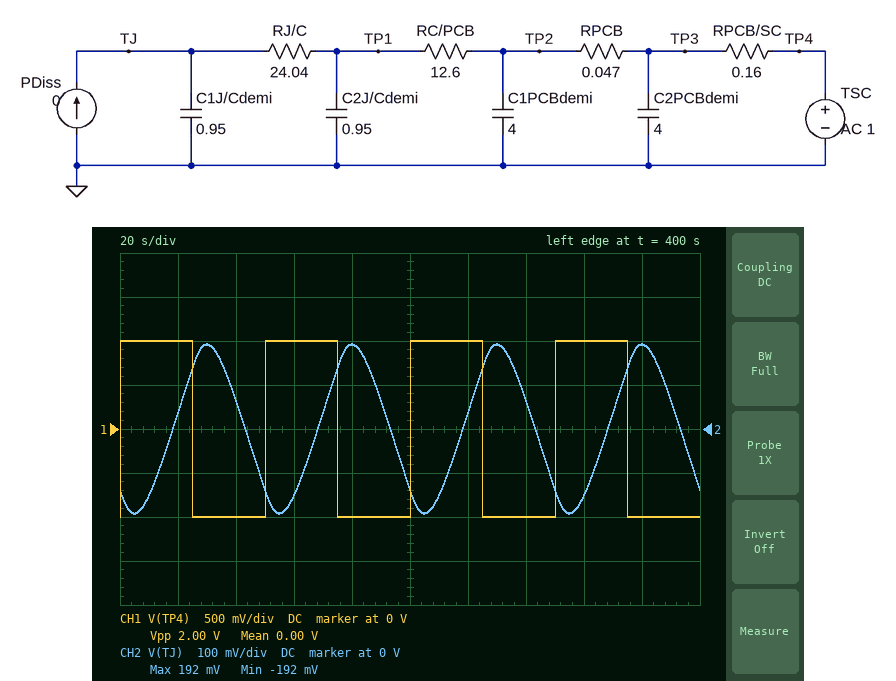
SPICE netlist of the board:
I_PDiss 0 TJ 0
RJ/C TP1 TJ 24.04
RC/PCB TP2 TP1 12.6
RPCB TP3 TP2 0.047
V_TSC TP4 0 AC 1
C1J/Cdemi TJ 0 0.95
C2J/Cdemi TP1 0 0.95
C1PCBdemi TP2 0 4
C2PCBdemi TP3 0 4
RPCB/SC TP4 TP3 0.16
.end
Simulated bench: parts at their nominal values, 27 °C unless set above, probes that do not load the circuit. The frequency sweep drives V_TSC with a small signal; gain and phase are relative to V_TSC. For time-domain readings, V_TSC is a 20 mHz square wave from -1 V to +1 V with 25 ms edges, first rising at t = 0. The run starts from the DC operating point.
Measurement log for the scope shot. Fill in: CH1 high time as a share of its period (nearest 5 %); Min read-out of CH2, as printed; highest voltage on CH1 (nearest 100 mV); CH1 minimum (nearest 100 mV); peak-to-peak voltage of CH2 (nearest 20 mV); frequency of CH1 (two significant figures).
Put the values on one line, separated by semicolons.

50 %; -192 mV; 1.0 V; -1.0 V; 380 mV; 20 mHz
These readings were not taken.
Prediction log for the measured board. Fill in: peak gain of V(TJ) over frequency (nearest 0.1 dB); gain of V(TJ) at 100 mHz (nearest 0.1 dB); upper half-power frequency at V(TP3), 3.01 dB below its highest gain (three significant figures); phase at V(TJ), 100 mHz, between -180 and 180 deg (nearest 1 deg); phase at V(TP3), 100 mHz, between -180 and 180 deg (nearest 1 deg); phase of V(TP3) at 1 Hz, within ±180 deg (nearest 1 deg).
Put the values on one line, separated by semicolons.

0 dB; -43.4 dB; 116 mHz; 152 deg; -37 deg; -62 deg
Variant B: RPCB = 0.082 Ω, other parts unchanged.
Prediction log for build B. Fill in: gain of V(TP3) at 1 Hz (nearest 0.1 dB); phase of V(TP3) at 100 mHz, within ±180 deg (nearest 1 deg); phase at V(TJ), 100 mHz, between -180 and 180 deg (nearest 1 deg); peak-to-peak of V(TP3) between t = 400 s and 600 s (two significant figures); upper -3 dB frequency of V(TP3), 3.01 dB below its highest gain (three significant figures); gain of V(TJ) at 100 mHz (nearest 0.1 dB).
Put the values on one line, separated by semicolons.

-14.7 dB; -36 deg; 148 deg; 2.0 V; 112 mHz; -43.7 dB
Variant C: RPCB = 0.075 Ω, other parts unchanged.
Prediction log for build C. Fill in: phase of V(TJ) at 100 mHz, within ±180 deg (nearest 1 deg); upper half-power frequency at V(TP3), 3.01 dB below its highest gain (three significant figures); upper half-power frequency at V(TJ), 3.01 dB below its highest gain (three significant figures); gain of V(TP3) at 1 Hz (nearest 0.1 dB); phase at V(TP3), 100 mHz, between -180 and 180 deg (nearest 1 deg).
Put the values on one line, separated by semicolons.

149 deg; 113 mHz; 3.83 mHz; -14.9 dB; -36 deg
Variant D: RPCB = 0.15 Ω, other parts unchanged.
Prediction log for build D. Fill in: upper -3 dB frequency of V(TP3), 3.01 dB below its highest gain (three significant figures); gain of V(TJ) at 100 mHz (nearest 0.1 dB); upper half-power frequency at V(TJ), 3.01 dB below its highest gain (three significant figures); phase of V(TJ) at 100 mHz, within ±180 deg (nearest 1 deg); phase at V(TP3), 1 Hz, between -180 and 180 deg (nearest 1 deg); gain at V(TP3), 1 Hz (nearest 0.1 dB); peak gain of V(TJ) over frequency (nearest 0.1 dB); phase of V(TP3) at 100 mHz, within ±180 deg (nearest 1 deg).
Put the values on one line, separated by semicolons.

109 mHz; -44.3 dB; 3.82 mHz; 142 deg; -65 deg; -13.5 dB; 0 dB; -33 deg
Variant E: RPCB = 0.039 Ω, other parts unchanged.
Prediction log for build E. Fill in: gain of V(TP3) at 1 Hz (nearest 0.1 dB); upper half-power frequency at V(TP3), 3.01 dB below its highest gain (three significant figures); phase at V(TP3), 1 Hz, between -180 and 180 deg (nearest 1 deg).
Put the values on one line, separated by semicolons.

-16.6 dB; 117 mHz; -64 deg
